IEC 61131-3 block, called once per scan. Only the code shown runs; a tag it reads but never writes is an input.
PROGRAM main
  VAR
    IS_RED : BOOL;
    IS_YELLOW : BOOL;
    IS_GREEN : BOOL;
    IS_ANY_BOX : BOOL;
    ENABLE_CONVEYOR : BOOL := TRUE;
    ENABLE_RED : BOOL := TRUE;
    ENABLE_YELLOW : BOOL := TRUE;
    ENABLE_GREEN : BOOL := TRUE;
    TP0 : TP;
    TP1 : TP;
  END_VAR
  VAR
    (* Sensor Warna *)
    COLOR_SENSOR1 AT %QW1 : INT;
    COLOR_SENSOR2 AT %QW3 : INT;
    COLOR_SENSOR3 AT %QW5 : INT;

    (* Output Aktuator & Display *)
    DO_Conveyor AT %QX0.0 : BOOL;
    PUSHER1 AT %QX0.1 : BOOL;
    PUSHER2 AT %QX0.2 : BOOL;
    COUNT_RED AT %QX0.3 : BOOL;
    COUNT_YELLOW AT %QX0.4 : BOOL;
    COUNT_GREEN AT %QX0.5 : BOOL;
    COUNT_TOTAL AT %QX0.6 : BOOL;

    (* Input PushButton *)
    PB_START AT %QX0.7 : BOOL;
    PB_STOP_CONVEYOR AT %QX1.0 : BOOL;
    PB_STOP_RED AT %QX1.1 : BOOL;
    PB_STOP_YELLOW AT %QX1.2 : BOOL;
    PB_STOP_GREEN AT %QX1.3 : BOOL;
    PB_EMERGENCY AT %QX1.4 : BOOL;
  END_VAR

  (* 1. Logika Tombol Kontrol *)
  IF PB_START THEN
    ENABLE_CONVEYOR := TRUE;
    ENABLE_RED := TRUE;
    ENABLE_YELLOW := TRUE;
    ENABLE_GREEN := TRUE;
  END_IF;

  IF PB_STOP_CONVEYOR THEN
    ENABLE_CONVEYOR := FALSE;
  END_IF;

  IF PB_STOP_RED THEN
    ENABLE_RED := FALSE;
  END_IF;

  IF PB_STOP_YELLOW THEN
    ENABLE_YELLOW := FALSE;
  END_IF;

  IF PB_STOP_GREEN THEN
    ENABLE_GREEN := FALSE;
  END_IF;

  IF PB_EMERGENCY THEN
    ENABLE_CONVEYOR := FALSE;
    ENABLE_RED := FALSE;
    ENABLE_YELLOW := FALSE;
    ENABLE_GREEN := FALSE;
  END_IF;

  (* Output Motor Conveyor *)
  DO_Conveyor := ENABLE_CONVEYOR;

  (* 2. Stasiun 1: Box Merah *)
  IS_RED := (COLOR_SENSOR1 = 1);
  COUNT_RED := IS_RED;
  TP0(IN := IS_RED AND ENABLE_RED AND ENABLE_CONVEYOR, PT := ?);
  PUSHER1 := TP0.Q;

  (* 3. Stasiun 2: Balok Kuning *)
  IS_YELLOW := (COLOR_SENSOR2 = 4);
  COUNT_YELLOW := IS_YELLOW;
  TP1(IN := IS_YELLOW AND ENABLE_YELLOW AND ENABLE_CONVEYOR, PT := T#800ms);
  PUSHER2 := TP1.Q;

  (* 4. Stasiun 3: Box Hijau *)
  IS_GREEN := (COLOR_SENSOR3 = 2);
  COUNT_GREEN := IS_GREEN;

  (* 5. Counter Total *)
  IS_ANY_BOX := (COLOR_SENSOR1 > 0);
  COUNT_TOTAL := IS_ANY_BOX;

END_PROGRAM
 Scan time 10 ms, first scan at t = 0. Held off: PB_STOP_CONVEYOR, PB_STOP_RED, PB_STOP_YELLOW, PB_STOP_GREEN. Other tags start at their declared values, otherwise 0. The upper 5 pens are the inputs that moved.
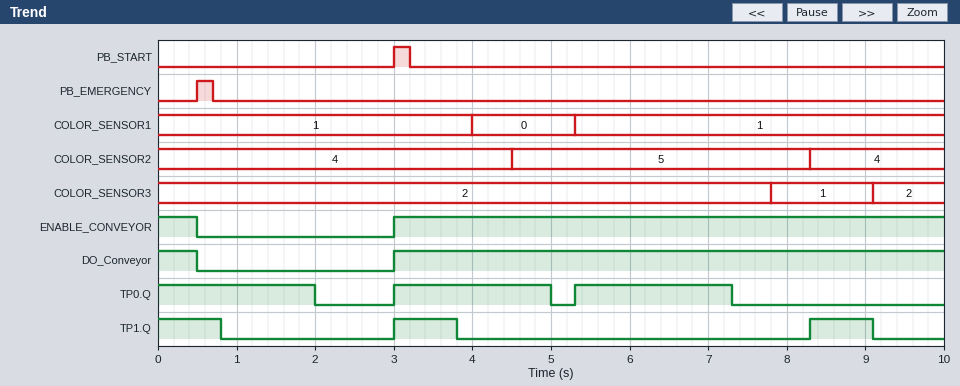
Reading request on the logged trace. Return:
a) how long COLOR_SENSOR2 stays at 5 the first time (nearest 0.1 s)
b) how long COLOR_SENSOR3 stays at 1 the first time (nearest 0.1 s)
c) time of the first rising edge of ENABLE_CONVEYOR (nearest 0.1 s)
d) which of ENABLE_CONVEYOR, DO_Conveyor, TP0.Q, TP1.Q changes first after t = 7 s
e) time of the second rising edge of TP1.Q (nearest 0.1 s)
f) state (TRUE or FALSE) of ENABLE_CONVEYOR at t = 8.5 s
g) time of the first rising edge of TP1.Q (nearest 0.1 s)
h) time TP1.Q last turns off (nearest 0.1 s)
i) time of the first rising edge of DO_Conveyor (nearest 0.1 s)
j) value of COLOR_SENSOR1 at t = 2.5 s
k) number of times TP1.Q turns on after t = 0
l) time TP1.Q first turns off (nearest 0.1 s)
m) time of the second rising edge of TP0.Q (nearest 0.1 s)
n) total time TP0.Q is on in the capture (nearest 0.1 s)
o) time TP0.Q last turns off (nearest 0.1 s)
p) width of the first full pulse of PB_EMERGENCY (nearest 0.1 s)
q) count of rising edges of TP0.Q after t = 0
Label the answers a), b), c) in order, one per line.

a) 3.8 s
b) 1.3 s
c) 3.0 s
d) TP0.Q
e) 8.3 s
f) TRUE
g) 3.0 s
h) 9.1 s
i) 3.0 s
j) 1
k) 2
l) 0.8 s
m) 5.3 s
n) 6.0 s
o) 7.3 s
p) 0.2 s
q) 2
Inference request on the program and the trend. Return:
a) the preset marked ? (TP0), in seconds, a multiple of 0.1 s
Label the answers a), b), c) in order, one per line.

a) 2.0 s
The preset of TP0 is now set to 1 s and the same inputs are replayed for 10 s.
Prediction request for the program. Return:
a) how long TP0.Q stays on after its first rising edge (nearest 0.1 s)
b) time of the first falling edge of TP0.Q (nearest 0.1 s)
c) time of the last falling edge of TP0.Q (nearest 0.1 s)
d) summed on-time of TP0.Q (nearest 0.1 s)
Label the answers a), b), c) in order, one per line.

a) 1.0 s
b) 1.0 s
c) 6.3 s
d) 3.0 s
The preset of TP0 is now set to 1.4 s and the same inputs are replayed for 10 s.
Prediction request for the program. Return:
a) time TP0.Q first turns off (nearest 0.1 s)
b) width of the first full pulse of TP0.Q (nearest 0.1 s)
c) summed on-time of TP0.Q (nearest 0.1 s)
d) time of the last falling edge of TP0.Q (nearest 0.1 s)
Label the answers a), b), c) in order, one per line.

a) 1.4 s
b) 1.4 s
c) 4.2 s
d) 6.7 s
